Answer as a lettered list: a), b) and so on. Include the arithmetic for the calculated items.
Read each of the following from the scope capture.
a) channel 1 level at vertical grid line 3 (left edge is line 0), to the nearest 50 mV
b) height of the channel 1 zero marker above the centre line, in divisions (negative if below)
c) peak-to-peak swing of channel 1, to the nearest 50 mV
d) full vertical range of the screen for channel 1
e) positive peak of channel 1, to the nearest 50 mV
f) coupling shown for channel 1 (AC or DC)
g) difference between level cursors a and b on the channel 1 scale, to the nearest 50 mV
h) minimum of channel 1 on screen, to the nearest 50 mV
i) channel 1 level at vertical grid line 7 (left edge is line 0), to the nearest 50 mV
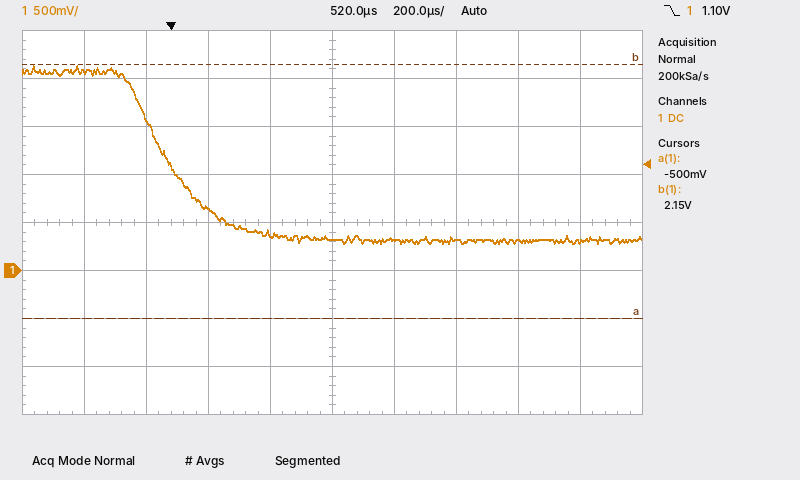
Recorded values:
a) 650 mV
b) -1.0 div
c) 2.15 V − (300 mV) = 1.85 V
d) 4 V
e) 2.15 V
f) DC
g) 2.65 V
h) 300 mV
i) 300 mV
